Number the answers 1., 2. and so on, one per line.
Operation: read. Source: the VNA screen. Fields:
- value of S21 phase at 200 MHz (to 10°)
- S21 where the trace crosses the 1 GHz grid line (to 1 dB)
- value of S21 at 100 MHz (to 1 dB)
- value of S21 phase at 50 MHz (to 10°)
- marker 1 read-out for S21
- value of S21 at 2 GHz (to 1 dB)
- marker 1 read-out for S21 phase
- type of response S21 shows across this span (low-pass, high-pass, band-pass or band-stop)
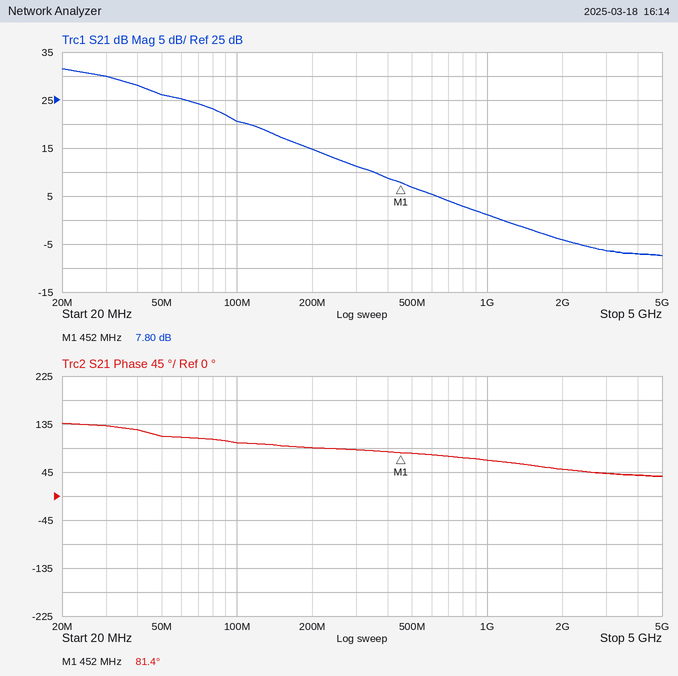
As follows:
1. 90°
2. 1 dB
3. 21 dB
4. 110°
5. 7.80 dB
6. -4 dB
7. 81.4°
8. low-pass
